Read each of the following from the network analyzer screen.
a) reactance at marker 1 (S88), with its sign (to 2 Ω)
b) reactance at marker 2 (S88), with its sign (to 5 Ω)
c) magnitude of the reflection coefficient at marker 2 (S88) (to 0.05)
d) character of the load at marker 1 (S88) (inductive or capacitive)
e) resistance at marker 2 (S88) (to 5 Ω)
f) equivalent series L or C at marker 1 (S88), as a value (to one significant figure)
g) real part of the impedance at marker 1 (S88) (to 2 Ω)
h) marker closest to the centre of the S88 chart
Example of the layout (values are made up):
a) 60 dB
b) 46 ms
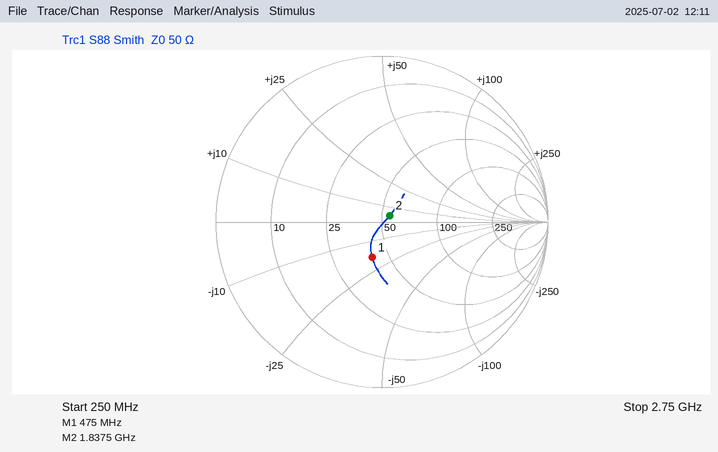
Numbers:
a) -18 Ω
b) +5 Ω
c) 0.05
d) capacitive
e) 55 Ω
f) 20 pF
g) 40 Ω
h) marker 2
